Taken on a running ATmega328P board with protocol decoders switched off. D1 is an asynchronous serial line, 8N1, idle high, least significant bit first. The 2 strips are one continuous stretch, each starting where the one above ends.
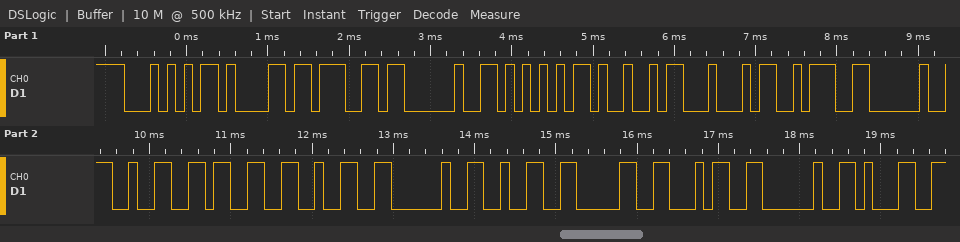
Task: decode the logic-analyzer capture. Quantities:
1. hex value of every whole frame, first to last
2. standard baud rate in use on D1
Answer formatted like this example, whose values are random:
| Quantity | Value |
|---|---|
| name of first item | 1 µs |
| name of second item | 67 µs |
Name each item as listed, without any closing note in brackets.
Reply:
| Quantity | Value |
|---|---|
| hex value of every whole frame, first to last | 0x54 0x61 0x67 0x20 0x55 0x49 0x44 0x3A 0x20 0x32 0x33 0x32 0x20 0x32 0x30 0x34 0x20 0x31 |
| standard baud rate in use on D1 | 9600 baud |
